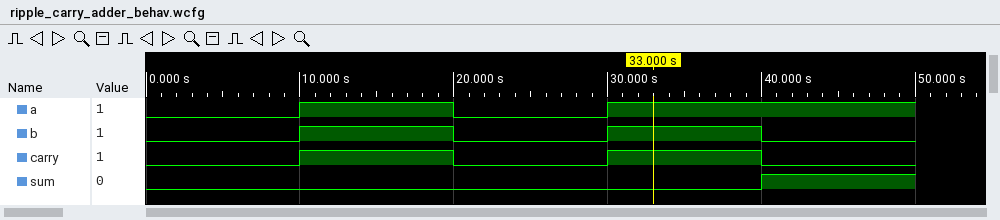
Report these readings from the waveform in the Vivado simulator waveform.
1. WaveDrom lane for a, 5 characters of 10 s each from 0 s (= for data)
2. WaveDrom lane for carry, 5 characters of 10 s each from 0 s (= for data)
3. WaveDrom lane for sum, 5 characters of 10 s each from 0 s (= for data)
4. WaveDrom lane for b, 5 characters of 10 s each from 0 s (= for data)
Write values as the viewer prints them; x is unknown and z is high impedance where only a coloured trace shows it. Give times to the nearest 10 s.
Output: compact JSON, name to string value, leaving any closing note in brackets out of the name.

{"WaveDrom lane for a, 5 characters of 10 s each from 0 s": "{name: 'a', wave: '0101.'}", "WaveDrom lane for carry, 5 characters of 10 s each from 0 s": "{name: 'carry', wave: '01010'}", "WaveDrom lane for sum, 5 characters of 10 s each from 0 s": "{name: 'sum', wave: '0...1'}", "WaveDrom lane for b, 5 characters of 10 s each from 0 s": "{name: 'b', wave: '01010'}"}
